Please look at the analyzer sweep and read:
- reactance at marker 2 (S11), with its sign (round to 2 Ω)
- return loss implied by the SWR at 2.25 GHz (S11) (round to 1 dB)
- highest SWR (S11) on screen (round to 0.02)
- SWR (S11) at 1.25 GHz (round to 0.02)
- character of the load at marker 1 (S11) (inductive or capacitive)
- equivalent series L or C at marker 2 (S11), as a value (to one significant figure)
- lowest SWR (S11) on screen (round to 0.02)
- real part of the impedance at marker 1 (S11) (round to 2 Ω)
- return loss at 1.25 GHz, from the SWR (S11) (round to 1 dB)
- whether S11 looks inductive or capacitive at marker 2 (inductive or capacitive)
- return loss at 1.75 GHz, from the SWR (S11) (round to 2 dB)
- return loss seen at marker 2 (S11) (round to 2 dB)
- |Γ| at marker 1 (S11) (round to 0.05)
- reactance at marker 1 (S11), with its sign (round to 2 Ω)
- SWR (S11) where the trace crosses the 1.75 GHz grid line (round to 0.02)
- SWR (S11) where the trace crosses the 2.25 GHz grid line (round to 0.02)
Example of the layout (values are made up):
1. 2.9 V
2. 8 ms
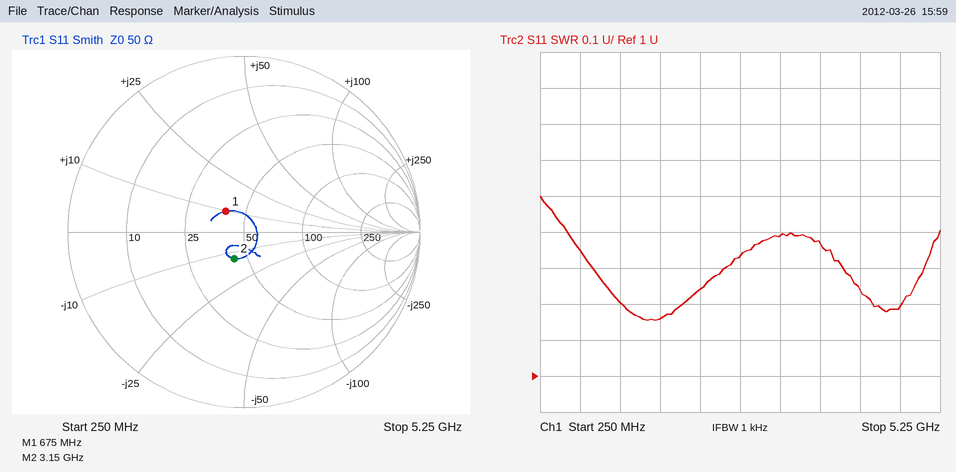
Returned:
1. -14 Ω
2. 19 dB
3. 1.50
4. 1.20
5. inductive
6. 4 pF
7. 1.16
8. 40 Ω
9. 21 dB
10. capacitive
11. 22 dB
12. 16 dB
13. 0.15
14. +10 Ω
15. 1.16
16. 1.24
